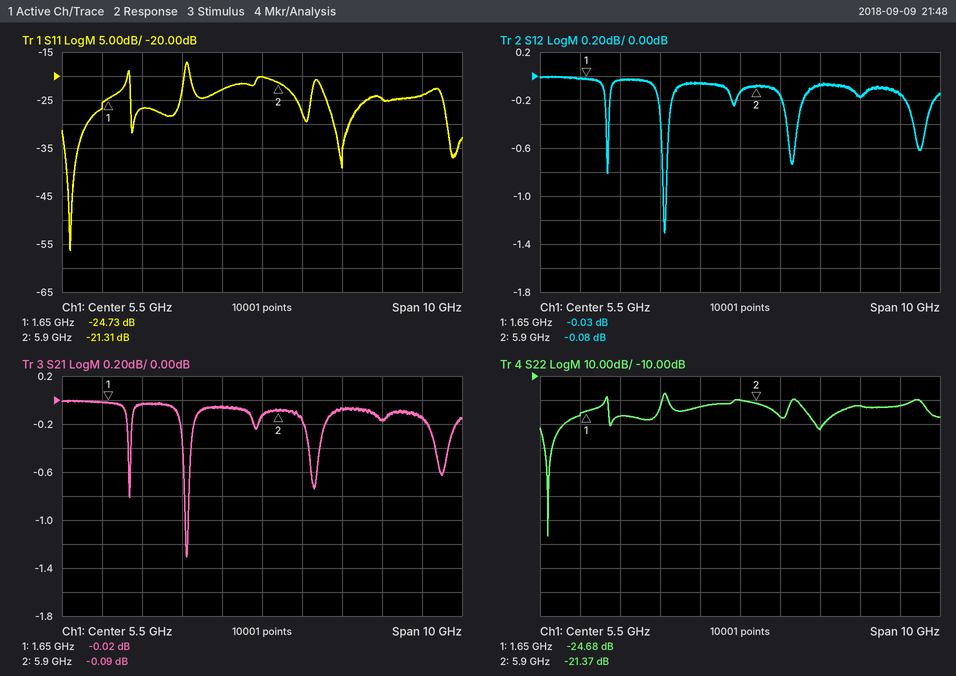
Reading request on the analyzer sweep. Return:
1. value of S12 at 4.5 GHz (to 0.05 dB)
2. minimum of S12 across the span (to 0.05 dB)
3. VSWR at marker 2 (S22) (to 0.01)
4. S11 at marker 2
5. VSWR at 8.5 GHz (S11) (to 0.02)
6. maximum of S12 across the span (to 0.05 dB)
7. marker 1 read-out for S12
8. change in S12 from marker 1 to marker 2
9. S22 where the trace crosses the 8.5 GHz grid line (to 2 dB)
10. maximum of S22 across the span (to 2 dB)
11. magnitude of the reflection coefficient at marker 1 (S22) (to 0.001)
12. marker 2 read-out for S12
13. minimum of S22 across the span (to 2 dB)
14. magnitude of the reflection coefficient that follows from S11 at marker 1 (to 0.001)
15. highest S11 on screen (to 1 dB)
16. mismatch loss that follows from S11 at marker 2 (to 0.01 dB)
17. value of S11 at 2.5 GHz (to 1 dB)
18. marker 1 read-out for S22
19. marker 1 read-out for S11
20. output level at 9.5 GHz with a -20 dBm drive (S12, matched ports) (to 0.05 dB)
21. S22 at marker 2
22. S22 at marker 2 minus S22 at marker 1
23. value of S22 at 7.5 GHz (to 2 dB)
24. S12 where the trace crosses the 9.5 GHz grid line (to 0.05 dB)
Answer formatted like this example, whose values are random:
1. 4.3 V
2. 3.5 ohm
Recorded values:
1. -0.05 dB
2. -1.30 dB
3. 1.19
4. -21.31 dB
5. 1.12
6. 0.00 dB
7. -0.03 dB
8. -0.05 dB
9. -22 dB
10. -18 dB
11. 0.058
12. -0.08 dB
13. -76 dB
14. 0.058
15. -17 dB
16. 0.03 dB
17. -27 dB
18. -24.68 dB
19. -24.73 dB
20. -20.15 dBm
21. -21.37 dB
22. 3.31 dB
23. -32 dB
24. -0.15 dB
